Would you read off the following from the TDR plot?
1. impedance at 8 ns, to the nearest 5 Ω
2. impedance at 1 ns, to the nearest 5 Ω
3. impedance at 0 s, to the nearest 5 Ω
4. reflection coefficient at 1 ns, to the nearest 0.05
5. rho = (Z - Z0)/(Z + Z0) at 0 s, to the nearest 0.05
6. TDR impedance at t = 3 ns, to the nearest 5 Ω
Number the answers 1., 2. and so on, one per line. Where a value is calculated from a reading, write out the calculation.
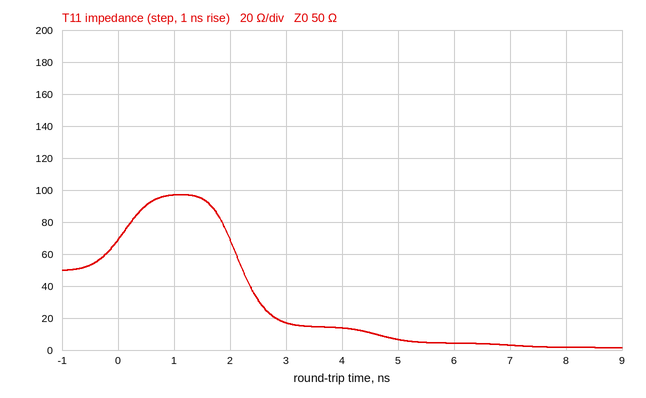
1. 0 Ω
2. 95 Ω
3. 70 Ω
4. (95 − 50)/(95 + 50) ≈ +0.310, so +0.30 to the nearest 0.05
5. (70 − 50)/(70 + 50) ≈ +0.167, so +0.15 to the nearest 0.05
6. 15 Ω
